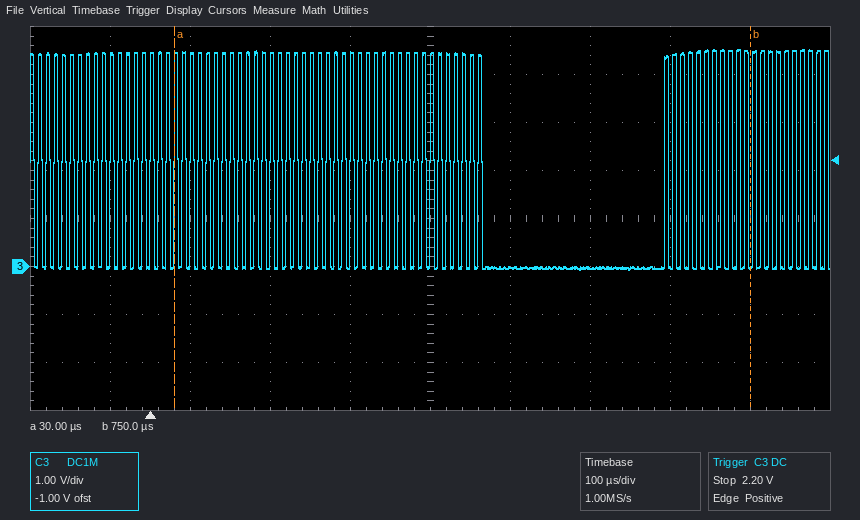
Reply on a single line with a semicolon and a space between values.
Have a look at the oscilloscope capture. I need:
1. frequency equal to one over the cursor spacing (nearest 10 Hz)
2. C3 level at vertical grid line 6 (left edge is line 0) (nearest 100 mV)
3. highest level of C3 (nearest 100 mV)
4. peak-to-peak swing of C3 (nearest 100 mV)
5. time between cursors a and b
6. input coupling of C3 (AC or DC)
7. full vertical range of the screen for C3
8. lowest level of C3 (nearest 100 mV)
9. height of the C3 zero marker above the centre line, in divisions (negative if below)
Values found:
1.39 kHz; 0.0 V; 4.5 V; 4.6 V; 720 µs; DC; 8 V; -100 mV; -1.0 div
